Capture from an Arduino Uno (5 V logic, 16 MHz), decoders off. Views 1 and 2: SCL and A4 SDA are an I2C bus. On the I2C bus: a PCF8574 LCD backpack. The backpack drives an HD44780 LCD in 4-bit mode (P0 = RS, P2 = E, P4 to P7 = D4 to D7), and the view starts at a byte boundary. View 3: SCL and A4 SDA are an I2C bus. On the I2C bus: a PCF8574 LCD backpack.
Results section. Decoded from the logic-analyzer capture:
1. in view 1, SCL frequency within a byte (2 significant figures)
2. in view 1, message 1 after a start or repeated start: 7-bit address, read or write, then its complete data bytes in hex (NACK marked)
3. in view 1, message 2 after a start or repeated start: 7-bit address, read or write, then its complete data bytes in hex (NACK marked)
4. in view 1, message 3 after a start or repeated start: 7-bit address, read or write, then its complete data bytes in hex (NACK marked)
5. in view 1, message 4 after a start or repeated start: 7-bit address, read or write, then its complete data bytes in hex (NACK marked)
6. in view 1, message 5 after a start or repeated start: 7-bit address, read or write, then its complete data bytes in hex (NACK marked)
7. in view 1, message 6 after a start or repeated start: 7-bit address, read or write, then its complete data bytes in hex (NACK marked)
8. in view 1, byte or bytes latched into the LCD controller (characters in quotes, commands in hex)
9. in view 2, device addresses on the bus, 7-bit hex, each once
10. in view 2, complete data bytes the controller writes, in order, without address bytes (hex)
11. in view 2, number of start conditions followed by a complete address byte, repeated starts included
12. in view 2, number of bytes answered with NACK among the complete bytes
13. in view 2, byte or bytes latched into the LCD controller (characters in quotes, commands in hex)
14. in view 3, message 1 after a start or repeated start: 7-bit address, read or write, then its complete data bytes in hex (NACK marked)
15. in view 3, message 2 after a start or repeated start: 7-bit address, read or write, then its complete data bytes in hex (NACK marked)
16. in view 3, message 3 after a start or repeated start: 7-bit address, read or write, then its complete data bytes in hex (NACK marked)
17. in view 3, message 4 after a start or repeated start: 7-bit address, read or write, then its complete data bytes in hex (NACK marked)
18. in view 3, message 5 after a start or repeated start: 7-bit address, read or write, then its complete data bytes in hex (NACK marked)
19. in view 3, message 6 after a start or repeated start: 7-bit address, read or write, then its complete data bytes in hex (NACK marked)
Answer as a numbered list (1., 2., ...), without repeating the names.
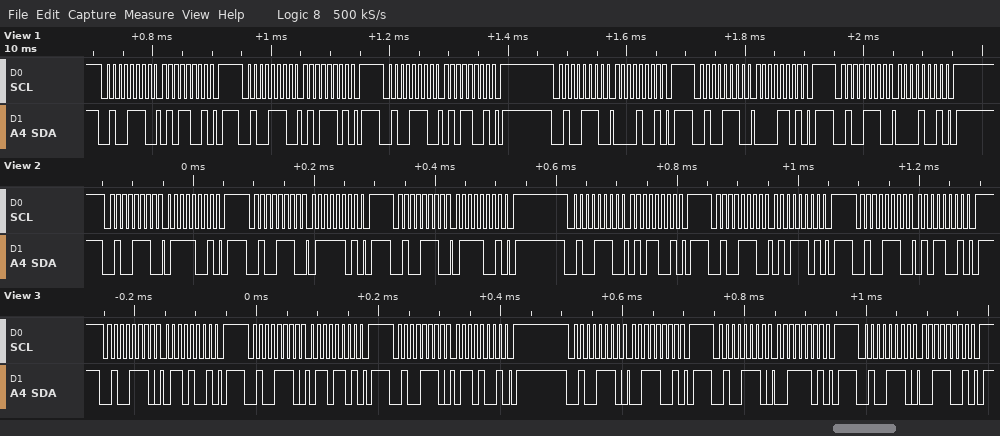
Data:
1. 100 kHz
2. 0x27 write: 59
3. 0x27 write: 5D
4. 0x27 write: 59
5. 0x27 write: 09
6. 0x27 write: 0D
7. 0x27 write: 09
8. 'P'
9. 0x27
10. 79 7D 79 59 5D 59
11. 6
12. 0
13. 'u'
14. 0x27 write: 69
15. 0x27 write: 6D
16. 0x27 write: 69
17. 0x27 write: 39
18. 0x27 write: 3D
19. 0x27 write: 39
